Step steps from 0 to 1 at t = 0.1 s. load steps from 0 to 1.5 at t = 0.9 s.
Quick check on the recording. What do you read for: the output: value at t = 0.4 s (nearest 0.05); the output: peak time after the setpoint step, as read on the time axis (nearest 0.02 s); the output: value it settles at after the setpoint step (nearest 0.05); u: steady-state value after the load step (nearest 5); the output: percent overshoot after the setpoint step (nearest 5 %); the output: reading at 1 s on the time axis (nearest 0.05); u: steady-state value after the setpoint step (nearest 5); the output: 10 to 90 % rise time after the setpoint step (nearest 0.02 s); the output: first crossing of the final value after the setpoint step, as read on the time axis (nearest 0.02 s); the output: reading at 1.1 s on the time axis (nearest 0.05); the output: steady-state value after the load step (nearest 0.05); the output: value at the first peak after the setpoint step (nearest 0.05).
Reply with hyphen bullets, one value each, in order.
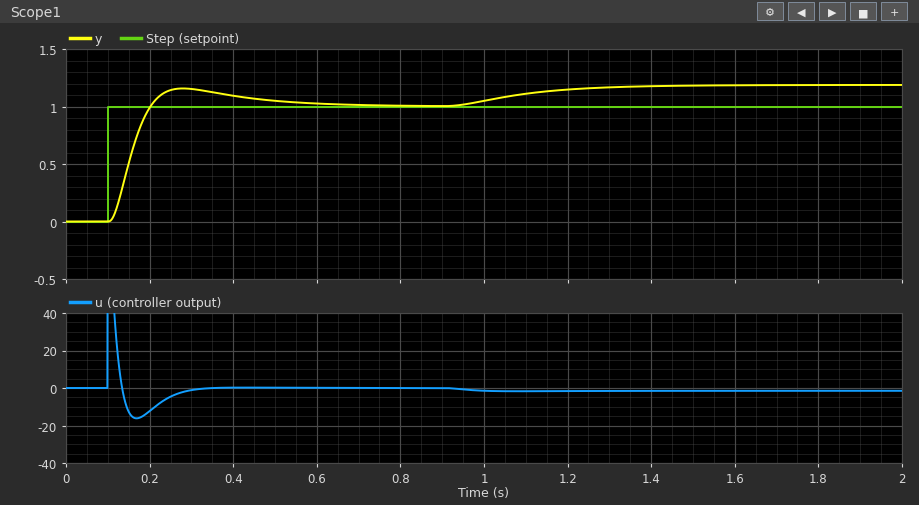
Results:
- 1.10
- 0.28 s
- 1.00
- 0
- 15 %
- 1.05
- 0
- 0.06 s
- 0.20 s
- 1.10
- 1.20
- 1.15
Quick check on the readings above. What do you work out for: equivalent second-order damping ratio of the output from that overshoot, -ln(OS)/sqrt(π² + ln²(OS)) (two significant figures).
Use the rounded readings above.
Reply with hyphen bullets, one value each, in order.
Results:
- 0.52
